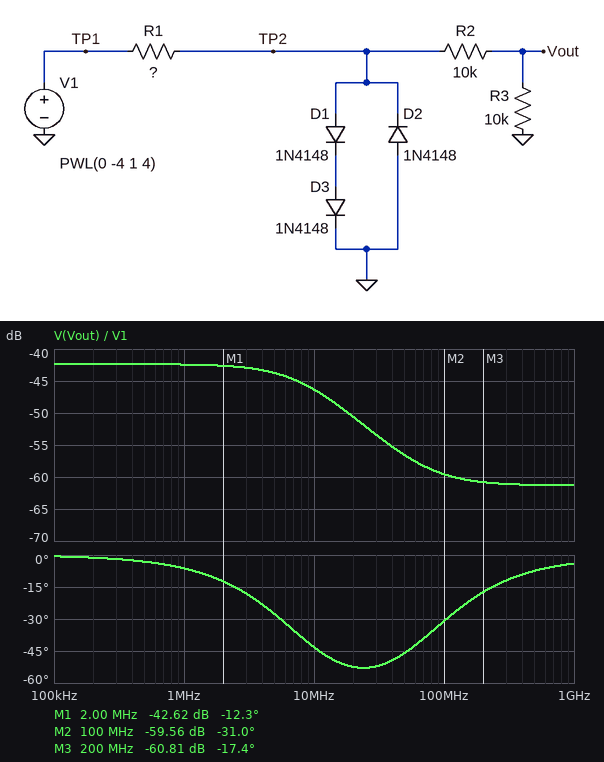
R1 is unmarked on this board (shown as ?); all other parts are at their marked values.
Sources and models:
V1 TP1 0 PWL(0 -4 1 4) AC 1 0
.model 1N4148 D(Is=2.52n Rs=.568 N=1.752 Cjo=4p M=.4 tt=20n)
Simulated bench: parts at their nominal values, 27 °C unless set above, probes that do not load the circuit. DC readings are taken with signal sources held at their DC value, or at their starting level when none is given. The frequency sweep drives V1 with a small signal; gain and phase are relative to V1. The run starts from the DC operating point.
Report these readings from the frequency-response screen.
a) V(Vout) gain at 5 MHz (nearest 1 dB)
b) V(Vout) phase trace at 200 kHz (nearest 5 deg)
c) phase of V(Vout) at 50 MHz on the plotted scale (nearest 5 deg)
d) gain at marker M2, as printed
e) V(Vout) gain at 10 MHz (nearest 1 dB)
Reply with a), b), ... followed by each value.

a) -44 dB
b) 0 deg
c) -45 deg
d) -59.56 dB
e) -46 dB
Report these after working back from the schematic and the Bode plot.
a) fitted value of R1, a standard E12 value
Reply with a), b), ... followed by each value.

a) 330 Ω
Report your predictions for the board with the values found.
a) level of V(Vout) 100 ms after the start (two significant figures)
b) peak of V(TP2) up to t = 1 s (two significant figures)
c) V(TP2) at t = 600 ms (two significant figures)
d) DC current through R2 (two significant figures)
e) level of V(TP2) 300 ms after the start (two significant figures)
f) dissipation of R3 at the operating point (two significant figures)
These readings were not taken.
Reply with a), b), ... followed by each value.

a) -340 mV
b) 1.4 V
c) 780 mV
d) 35 µA
e) -630 mV
f) 12 µW
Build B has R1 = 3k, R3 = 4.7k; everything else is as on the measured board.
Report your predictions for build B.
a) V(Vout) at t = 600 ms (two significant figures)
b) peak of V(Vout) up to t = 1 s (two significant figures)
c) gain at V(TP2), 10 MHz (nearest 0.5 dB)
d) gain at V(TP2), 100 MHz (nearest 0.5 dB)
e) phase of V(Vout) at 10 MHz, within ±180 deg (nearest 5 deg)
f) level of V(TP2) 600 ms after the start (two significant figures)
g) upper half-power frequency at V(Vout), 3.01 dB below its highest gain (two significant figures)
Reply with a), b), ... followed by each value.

a) 210 mV
b) 370 mV
c) -41.5 dB
d) -59.0 dB
e) -50 deg
f) 660 mV
g) 8.0 MHz
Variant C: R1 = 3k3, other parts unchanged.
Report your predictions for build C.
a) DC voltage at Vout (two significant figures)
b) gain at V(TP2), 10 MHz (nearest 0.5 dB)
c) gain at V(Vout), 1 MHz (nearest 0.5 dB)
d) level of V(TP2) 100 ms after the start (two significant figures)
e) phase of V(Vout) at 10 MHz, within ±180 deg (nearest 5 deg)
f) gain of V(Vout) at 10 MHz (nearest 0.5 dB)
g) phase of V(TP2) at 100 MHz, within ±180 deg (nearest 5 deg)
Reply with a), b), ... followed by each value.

a) -290 mV
b) -41.5 dB
c) -43.5 dB
d) -570 mV
e) -50 deg
f) -47.5 dB
g) -75 deg
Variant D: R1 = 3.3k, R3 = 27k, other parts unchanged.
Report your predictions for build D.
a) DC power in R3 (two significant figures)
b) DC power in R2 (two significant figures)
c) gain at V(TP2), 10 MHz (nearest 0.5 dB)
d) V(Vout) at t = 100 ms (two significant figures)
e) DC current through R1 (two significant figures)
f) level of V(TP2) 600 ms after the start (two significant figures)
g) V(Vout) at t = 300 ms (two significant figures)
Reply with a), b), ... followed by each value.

a) 6.8 µW
b) 2.5 µW
c) -41.5 dB
d) -420 mV
e) 1.0 mA
f) 710 mV
g) -390 mV
